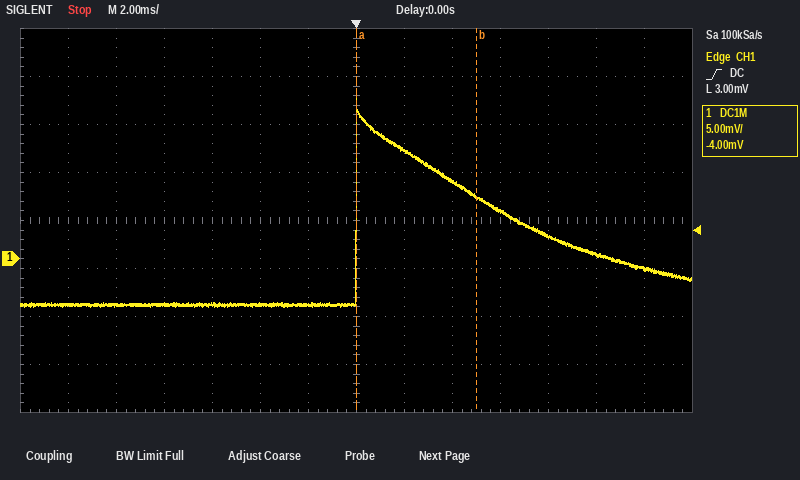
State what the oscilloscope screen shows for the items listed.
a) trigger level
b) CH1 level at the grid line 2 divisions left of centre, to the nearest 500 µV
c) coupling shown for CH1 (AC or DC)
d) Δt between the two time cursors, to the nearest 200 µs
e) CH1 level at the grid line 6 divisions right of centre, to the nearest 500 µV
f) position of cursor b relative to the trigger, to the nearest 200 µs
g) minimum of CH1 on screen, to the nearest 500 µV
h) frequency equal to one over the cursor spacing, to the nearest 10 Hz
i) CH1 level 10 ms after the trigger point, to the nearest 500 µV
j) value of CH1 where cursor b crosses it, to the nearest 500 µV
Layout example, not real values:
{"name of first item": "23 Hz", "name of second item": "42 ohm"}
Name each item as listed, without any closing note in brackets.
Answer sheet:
{"trigger level": "3.00 mV", "CH1 level at the grid line 2 divisions left of centre, to the nearest 500 µV": "-4.5 mV", "coupling shown for CH1": "DC", "Δt between the two time cursors, to the nearest 200 µs": "5.0 ms", "CH1 level at the grid line 6 divisions right of centre, to the nearest 500 µV": "-1.0 mV", "position of cursor b relative to the trigger, to the nearest 200 µs": "+5.0 ms", "minimum of CH1 on screen, to the nearest 500 µV": "-5.0 mV", "frequency equal to one over the cursor spacing, to the nearest 10 Hz": "200 Hz", "CH1 level 10 ms after the trigger point, to the nearest 500 µV": "500 µV", "value of CH1 where cursor b crosses it, to the nearest 500 µV": "6.5 mV"}
